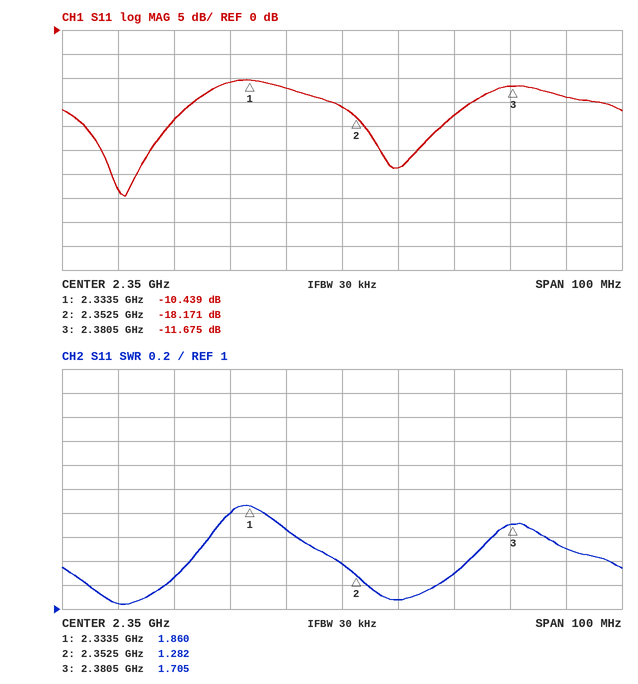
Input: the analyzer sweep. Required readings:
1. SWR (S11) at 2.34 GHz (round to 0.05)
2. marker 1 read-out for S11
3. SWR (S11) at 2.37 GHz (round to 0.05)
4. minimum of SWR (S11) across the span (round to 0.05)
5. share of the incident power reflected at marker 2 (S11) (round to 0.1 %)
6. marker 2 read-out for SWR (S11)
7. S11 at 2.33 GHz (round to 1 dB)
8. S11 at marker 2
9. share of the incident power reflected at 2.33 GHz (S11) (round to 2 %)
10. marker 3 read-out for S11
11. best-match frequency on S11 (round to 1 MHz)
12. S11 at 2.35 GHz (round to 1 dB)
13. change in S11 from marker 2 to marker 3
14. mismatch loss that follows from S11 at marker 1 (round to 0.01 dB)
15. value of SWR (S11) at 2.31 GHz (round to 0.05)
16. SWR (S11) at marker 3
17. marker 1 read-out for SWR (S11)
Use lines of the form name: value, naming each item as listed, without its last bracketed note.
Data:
SWR (S11) at 2.34 GHz: 1.65
marker 1 read-out for S11: -10.439 dB
SWR (S11) at 2.37 GHz: 1.30
minimum of SWR (S11) across the span: 1.05
share of the incident power reflected at marker 2 (S11): 1.5 %
marker 2 read-out for SWR: 1.282
S11 at 2.33 GHz: -11 dB
S11 at marker 2: -18.171 dB
share of the incident power reflected at 2.33 GHz (S11): 8 %
marker 3 read-out for S11: -11.675 dB
best-match frequency on S11: 2.311 GHz
S11 at 2.35 GHz: -16 dB
change in S11 from marker 2 to marker 3: 6.496 dB
mismatch loss that follows from S11 at marker 1: 0.41 dB
value of SWR (S11) at 2.31 GHz: 1.05
SWR (S11) at marker 3: 1.705
marker 1 read-out for SWR: 1.860
